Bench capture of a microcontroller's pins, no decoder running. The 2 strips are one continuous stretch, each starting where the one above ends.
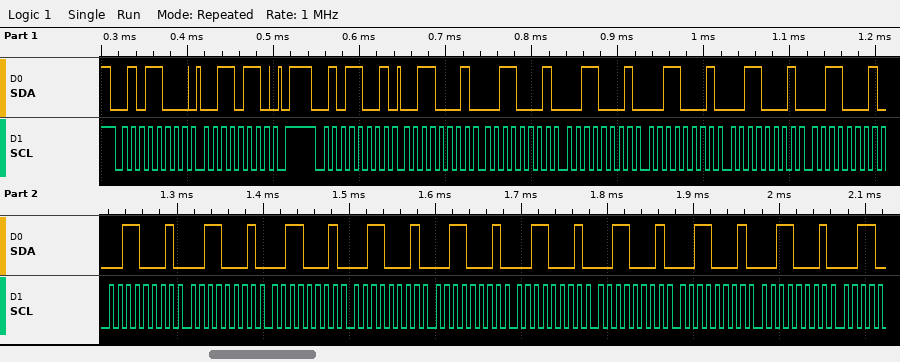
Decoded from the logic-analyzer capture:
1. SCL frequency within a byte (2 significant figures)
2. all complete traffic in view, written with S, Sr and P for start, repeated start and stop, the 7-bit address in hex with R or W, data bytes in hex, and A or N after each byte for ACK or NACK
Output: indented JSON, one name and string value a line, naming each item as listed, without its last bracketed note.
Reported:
{
  "SCL frequency within a byte": "100 kHz",
  "all complete traffic in view, written with S, Sr and P for start, repeated start and stop, the 7-bit address in hex with R or W, data bytes in hex, and A or N after each byte for ACK or NACK": "S 2CW A 36 A P S 2CR A 31 A 31 A 31 A 31 A 31 A 31 A 31 A 31 A 31 A 31 A 31 A 31 A 31 A 31 A 31 A"
}
